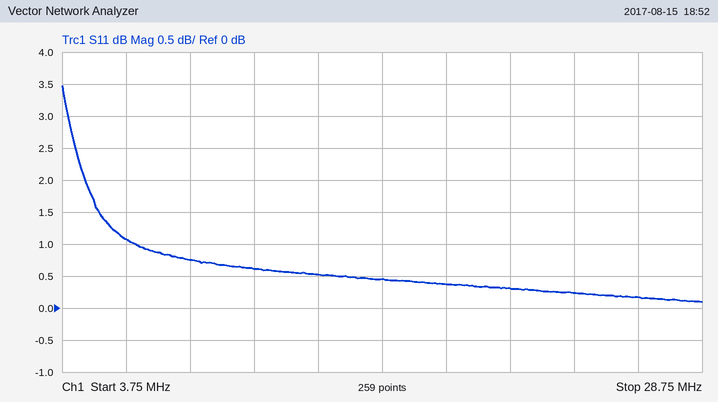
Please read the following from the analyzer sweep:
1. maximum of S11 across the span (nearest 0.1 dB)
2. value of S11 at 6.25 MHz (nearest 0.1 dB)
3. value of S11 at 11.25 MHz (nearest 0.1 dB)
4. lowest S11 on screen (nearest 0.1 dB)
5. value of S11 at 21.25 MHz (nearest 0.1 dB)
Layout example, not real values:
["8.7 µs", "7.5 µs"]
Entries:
["3.5 dB", "1.1 dB", "0.6 dB", "0.1 dB", "0.3 dB"]
